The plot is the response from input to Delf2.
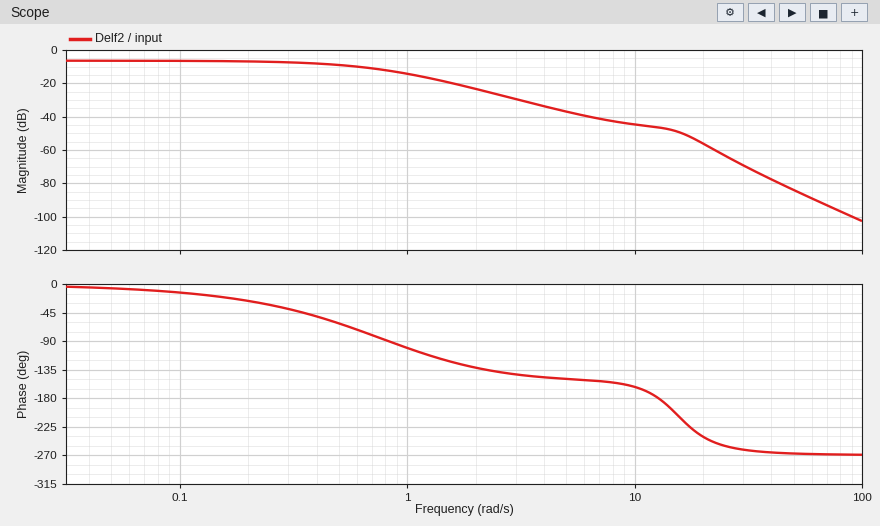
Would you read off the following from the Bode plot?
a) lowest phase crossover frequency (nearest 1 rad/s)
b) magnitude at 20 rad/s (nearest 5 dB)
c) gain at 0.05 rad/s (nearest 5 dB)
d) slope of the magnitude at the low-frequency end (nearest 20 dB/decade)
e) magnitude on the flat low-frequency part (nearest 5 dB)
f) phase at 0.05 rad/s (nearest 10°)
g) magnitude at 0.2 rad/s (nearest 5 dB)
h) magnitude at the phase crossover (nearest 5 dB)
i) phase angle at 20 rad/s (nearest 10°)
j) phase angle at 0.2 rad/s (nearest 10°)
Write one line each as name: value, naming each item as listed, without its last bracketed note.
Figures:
lowest phase crossover frequency: 13 rad/s
magnitude at 20 rad/s: -55 dB
gain at 0.05 rad/s: -5 dB
slope of the magnitude at the low-frequency end: 0 dB/decade
magnitude on the flat low-frequency part: -5 dB
phase at 0.05 rad/s: -10°
magnitude at 0.2 rad/s: -5 dB
magnitude at the phase crossover: -45 dB
phase angle at 20 rad/s: -240°
phase angle at 0.2 rad/s: -30°
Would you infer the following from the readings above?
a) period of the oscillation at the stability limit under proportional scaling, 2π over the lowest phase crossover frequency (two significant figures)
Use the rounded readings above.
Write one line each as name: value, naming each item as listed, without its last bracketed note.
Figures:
period of the oscillation at the stability limit under proportional scaling, 2π over the lowest phase crossover frequency: 0.48 s
